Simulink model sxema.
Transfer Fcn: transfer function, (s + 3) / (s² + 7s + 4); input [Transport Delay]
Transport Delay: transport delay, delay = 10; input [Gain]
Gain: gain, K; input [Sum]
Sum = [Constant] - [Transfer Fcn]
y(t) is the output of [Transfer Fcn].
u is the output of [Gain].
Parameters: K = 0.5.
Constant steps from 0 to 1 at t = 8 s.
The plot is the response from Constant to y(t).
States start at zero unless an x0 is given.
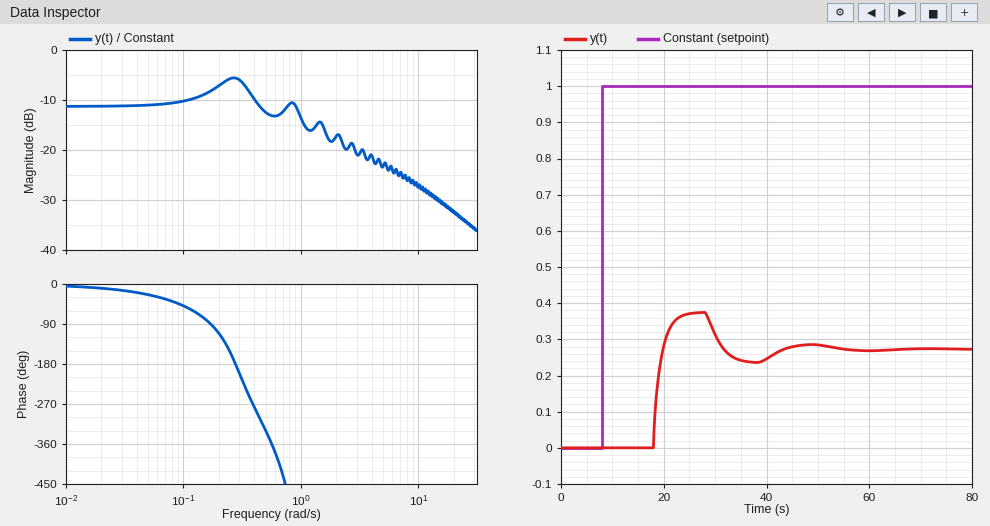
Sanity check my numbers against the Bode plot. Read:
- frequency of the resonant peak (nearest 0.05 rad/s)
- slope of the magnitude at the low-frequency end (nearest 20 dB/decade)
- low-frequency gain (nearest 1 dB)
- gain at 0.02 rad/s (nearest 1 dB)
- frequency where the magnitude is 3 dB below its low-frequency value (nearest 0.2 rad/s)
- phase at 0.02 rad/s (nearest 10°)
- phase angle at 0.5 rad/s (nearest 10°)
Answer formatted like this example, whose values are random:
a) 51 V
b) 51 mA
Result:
a) 0.25 rad/s
b) 0 dB/decade
c) -11 dB
d) -11 dB
e) 1.0 rad/s
f) -10°
g) -330°
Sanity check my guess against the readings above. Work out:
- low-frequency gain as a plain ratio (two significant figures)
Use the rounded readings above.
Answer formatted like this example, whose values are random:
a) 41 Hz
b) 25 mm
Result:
a) 0.28
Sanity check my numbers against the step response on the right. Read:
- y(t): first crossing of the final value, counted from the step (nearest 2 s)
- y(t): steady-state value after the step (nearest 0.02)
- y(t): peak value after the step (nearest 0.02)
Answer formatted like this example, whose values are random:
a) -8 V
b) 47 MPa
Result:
a) 12 s
b) 0.28
c) 0.38
